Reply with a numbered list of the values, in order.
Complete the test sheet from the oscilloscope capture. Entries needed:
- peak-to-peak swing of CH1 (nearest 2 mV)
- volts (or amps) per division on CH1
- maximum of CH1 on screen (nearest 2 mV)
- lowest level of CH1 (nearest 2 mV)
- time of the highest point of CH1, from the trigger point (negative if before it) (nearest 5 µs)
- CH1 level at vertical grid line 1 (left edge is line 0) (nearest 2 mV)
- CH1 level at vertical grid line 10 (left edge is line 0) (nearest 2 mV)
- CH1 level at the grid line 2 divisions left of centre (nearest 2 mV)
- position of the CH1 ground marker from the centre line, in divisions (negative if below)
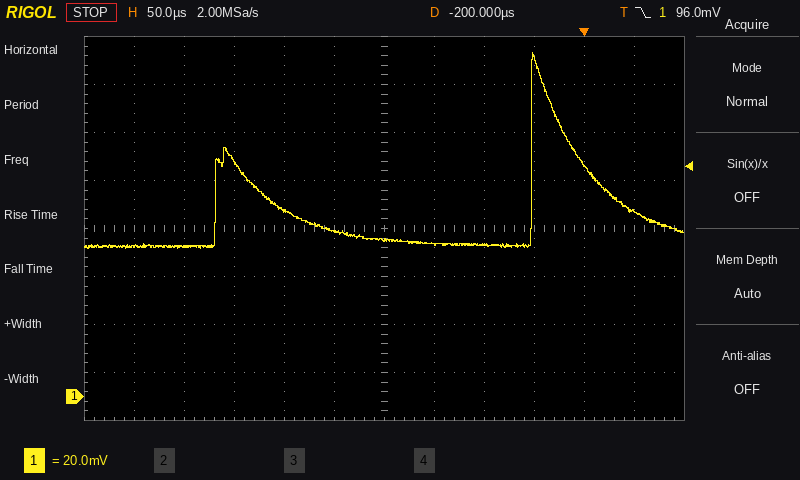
1. 82 mV
2. 20 mV
3. 144 mV
4. 62 mV
5. -50 µs
6. 62 mV
7. 96 mV
8. 78 mV
9. -3.5 div
